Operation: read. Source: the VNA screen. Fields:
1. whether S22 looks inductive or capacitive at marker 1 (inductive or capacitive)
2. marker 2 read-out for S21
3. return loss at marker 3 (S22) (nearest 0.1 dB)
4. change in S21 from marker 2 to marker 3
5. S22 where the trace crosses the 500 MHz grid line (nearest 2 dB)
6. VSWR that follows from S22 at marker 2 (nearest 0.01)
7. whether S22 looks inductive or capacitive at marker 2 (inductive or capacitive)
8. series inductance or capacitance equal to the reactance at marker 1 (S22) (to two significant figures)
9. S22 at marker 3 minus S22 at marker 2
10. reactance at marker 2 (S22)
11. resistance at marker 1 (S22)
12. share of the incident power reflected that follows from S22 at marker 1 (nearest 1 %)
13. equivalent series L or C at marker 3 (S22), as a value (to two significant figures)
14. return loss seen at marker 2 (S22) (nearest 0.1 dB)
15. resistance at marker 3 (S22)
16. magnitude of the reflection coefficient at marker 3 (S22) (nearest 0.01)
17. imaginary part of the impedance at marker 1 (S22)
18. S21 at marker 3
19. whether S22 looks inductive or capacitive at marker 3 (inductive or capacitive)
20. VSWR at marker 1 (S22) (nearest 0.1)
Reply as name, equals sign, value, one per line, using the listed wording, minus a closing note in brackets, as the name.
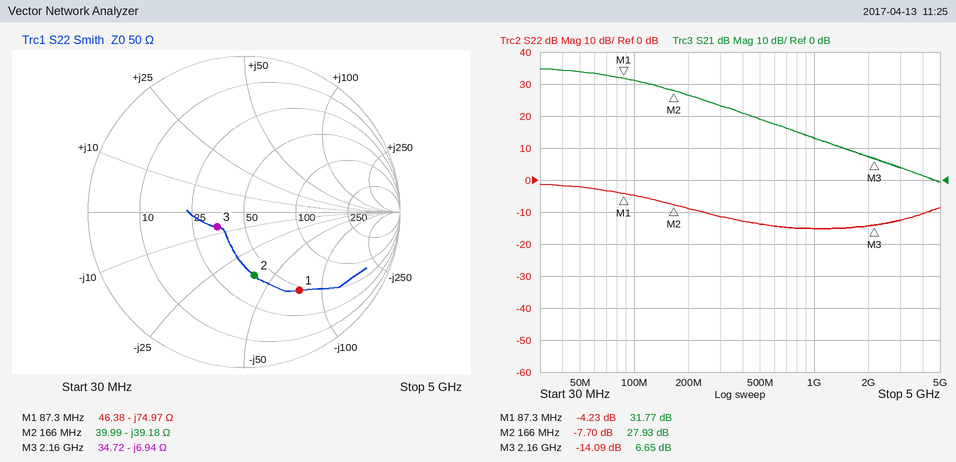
whether S22 looks inductive or capacitive at marker 1 = capacitive
marker 2 read-out for S21 = 27.93 dB
return loss at marker 3 (S22) = 14.1 dB
change in S21 from marker 2 to marker 3 = -21.28 dB
S22 where the trace crosses the 500 MHz grid line = -14 dB
VSWR that follows from S22 at marker 2 = 2.40
whether S22 looks inductive or capacitive at marker 2 = capacitive
series inductance or capacitance equal to the reactance at marker 1 (S22) = 24 pF
S22 at marker 3 minus S22 at marker 2 = -6.39 dB
reactance at marker 2 = -39.18 Ω
resistance at marker 1 = 46.38 Ω
share of the incident power reflected that follows from S22 at marker 1 = 38 %
equivalent series L or C at marker 3 (S22), as a value = 11 pF
return loss seen at marker 2 (S22) = 7.7 dB
resistance at marker 3 = 34.72 Ω
magnitude of the reflection coefficient at marker 3 (S22) = 0.20
imaginary part of the impedance at marker 1 = -74.97 Ω
S21 at marker 3 = 6.65 dB
whether S22 looks inductive or capacitive at marker 3 = capacitive
VSWR at marker 1 (S22) = 4.2
